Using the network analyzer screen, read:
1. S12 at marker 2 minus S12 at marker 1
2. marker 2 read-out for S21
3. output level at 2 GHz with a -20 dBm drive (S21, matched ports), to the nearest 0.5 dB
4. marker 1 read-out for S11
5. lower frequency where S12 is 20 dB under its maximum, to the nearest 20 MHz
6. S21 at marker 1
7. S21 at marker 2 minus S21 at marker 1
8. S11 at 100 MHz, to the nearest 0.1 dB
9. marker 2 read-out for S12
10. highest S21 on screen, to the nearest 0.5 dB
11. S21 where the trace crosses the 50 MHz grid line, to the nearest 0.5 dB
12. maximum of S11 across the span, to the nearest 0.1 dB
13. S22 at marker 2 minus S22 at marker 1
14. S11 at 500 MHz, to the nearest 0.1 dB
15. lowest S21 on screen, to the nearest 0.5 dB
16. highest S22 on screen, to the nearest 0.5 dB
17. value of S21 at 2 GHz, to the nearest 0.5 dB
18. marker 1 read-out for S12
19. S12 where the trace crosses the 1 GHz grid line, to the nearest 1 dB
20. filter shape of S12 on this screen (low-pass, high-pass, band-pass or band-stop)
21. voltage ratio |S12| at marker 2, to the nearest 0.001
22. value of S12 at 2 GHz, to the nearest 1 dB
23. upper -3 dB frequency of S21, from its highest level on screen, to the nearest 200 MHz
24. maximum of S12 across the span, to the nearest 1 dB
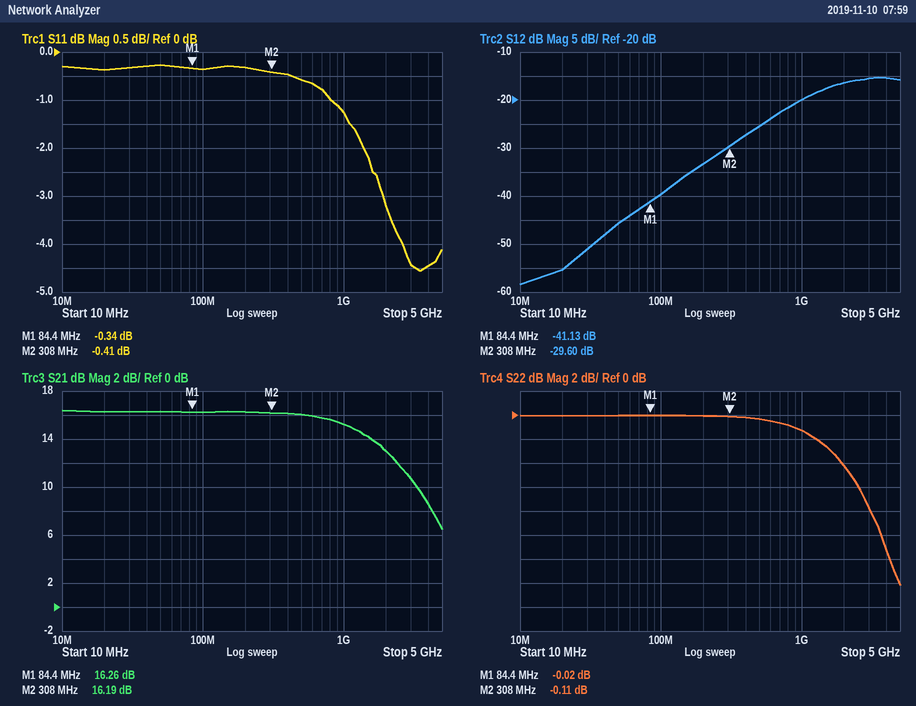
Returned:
11.53 dB
16.19 dB
-7.0 dBm
-0.34 dB
160 MHz
16.26 dB
-0.07 dB
-0.4 dB
-29.60 dB
16.5 dB
16.5 dB
-0.3 dB
-0.09 dB
-0.6 dB
6.5 dB
0.0 dB
13.0 dB
-41.13 dB
-20 dB
high-pass
0.033
-16 dB
1.8 GHz
-15 dB
